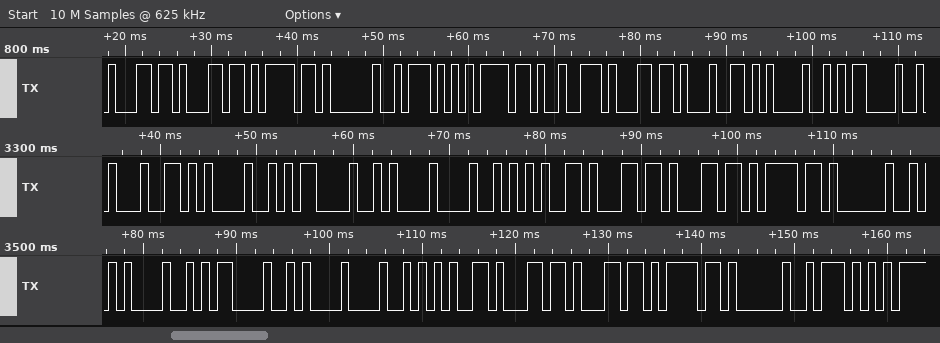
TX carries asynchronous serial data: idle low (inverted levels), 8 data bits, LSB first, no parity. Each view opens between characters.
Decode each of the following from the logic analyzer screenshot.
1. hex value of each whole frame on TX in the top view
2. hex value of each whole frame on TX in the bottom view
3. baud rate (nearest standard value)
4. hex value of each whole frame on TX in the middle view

27, 27, 21, BF, 51, 21, 1B, 27, 37, BD, E5
BD, E5, EB, 6F, 35, 27, 27, 21, BF, 51
1200 baud
37, BD, E5, EB, 6F, 35, 27, 27, 21, BF
